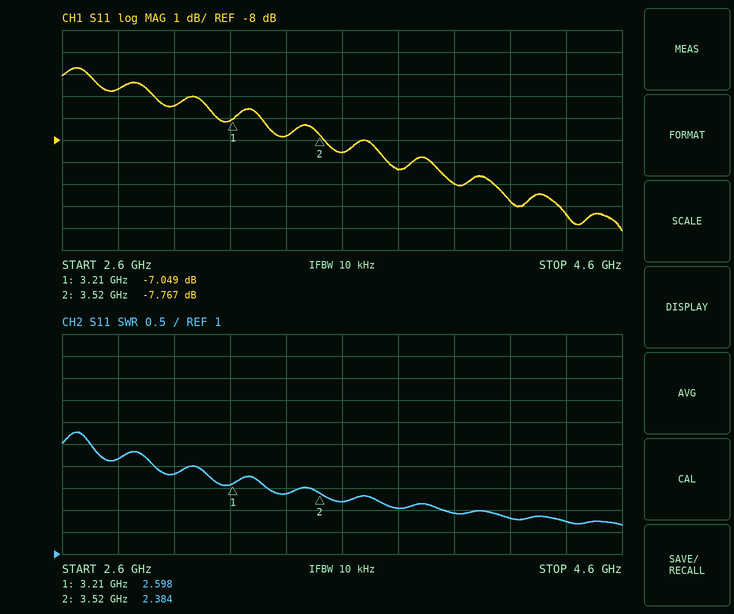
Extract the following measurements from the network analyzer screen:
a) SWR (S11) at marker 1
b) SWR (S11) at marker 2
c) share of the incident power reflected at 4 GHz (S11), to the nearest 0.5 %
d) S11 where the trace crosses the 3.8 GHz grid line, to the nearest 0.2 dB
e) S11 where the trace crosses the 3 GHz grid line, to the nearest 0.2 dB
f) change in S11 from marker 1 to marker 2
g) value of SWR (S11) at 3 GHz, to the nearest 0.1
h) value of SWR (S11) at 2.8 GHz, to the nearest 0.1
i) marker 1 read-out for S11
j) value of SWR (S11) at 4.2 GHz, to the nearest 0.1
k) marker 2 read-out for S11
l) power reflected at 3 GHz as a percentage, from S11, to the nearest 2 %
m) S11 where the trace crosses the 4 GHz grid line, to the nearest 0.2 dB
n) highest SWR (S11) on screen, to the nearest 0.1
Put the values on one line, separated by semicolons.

2.598; 2.384; 10.0 %; -9.4 dB; -6.4 dB; -0.718 dB; 2.8; 3.2; -7.049 dB; 1.8; -7.767 dB; 22 %; -10.0 dB; 3.8
